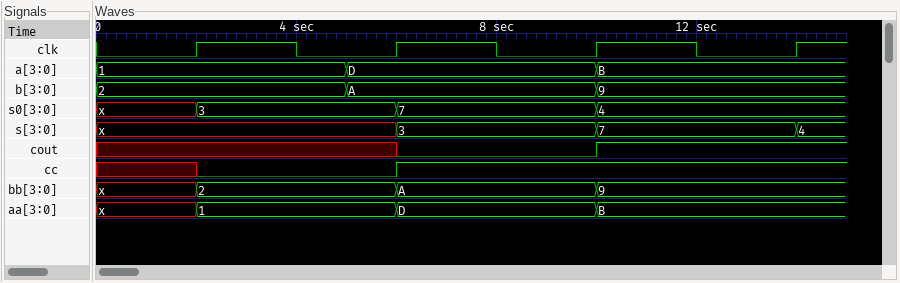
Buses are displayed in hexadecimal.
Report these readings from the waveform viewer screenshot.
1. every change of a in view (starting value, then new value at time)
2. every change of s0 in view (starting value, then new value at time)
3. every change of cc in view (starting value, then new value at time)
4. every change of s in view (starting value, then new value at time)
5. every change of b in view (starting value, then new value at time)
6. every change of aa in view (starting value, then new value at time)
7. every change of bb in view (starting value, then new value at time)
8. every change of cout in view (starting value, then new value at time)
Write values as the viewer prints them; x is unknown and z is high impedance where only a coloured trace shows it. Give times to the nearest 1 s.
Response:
1, D at 5 s, B at 10 s
x, 3 at 2 s, 7 at 6 s, 4 at 10 s
x, 0 at 2 s, 1 at 6 s
x, 3 at 6 s, 7 at 10 s, 4 at 14 s
2, A at 5 s, 9 at 10 s
x, 1 at 2 s, D at 6 s, B at 10 s
x, 2 at 2 s, A at 6 s, 9 at 10 s
x, 0 at 6 s, 1 at 10 s
